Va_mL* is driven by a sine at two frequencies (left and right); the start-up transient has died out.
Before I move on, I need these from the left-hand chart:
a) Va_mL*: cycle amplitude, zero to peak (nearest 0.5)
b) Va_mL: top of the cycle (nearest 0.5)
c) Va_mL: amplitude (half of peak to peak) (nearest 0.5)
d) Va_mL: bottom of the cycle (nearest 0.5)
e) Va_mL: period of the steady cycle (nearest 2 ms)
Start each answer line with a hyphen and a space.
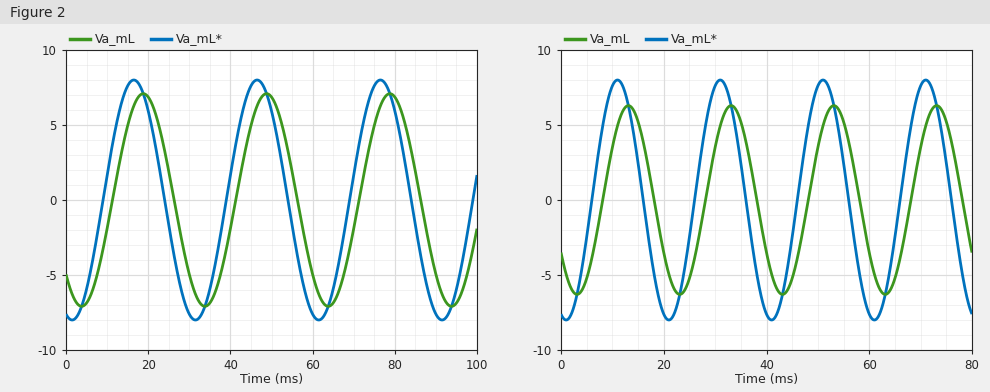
- 8.0
- 7.0
- 7.0
- -7.0
- 30 ms
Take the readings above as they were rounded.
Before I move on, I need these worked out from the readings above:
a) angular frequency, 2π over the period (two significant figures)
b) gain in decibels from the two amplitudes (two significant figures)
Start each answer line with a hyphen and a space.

- 0.21 rad/ms
- -1.2 dB
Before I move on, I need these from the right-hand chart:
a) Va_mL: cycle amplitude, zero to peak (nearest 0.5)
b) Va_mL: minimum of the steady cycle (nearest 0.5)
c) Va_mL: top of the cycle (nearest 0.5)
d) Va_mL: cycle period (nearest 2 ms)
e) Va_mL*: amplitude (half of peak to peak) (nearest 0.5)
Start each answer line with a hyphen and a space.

- 6.5
- -6.5
- 6.5
- 20 ms
- 8.0
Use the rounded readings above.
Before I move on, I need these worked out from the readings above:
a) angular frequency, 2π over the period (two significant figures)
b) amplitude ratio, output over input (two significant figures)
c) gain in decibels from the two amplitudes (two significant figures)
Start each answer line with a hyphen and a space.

- 0.31 rad/ms
- 0.81
- -1.8 dB
